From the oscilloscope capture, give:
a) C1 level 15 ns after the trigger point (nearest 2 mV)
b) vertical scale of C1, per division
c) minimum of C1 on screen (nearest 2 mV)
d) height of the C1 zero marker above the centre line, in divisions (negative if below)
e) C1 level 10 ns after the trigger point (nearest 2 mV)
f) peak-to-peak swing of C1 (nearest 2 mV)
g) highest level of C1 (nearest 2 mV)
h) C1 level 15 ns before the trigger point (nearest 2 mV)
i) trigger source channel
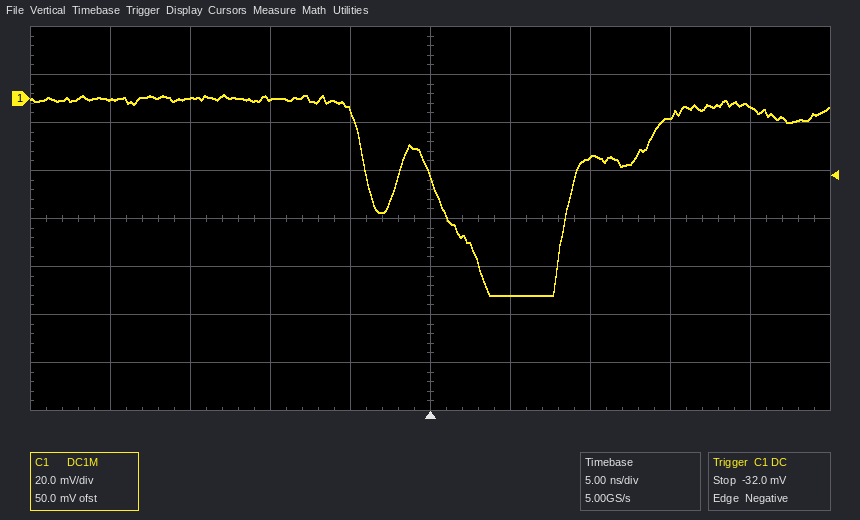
-8 mV
20 mV
-82 mV
+2.5 div
-24 mV
84 mV
2 mV
0 mV
C1
